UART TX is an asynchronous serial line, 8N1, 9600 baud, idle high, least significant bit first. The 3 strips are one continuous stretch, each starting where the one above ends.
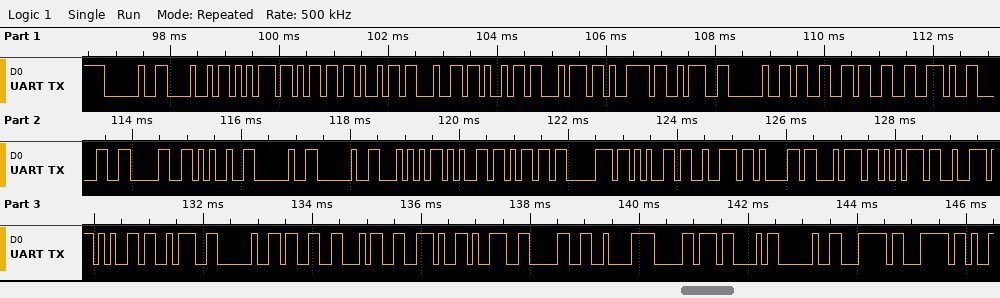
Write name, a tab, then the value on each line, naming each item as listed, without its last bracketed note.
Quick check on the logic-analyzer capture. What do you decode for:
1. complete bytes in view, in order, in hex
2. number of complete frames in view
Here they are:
complete bytes in view, in order, in hex	20 48 75 6D 69 64 69 74 79 3A 20 33 33 2E 30 30 25 20 20 54 65 6D 70 65 72 61 74 75 72 65 3A 20 33 34 2E 39 30 C2 B0 43 20 7C 7C
number of complete frames in view	43
